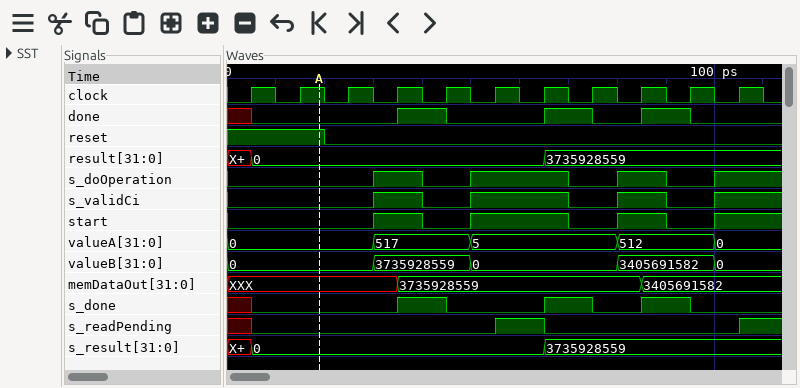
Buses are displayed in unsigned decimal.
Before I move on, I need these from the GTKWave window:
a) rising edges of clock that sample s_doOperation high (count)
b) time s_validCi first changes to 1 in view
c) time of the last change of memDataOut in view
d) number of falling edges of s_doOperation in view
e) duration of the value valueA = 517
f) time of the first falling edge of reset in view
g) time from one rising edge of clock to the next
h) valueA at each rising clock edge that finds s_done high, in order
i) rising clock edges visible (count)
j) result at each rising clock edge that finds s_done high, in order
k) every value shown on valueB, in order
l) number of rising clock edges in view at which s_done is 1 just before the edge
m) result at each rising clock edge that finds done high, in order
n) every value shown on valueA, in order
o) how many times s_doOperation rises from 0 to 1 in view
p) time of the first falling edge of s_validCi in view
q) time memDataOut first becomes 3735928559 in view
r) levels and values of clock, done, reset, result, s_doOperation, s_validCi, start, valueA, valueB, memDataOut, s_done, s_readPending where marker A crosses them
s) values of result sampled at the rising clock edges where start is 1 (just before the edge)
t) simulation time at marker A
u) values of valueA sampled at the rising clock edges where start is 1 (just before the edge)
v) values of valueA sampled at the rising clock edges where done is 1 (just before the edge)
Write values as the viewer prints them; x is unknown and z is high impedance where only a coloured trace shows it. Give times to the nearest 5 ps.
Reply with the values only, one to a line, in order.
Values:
5
30 ps
85 ps
3
20 ps
20 ps
10 ps
517, 5, 512
11
0, 3735928559, 3735928559
0, 3735928559, 0, 3405691582, 0
3
0, 3735928559, 3735928559
0, 517, 5, 512, 0
4
40 ps
35 ps
clock=1, done=0, reset=1, result=0, s_doOperation=0, s_validCi=0, start=0, valueA=0, valueB=0, memDataOut=XXX, s_done=0, s_readPending=0
0, 0, 0, 3735928559, 3735928559
20 ps
517, 5, 5, 512, 0
517, 5, 512
